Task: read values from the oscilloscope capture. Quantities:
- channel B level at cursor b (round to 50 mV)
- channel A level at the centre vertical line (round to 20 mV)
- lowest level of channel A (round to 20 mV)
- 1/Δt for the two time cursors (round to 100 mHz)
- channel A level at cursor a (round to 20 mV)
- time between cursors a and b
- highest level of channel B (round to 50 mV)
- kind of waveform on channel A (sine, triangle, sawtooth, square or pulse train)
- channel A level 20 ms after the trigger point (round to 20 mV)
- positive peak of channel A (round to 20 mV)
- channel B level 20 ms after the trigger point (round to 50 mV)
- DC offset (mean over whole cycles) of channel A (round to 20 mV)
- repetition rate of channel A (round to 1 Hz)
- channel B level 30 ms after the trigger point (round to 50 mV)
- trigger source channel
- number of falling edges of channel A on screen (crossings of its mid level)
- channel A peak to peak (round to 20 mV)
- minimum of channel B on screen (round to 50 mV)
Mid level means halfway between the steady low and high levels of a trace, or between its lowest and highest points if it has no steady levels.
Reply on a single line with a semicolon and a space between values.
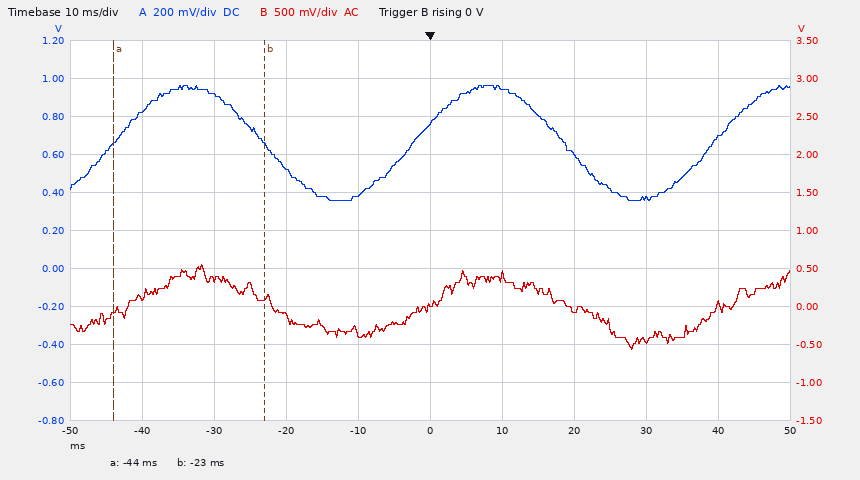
100 mV; 760 mV; 360 mV; 47.6 Hz; 660 mV; 21 ms; 550 mV; sine; 600 mV; 960 mV; -50 mV; 660 mV; 24 Hz; -450 mV; channel B; 2; 600 mV; -550 mV
